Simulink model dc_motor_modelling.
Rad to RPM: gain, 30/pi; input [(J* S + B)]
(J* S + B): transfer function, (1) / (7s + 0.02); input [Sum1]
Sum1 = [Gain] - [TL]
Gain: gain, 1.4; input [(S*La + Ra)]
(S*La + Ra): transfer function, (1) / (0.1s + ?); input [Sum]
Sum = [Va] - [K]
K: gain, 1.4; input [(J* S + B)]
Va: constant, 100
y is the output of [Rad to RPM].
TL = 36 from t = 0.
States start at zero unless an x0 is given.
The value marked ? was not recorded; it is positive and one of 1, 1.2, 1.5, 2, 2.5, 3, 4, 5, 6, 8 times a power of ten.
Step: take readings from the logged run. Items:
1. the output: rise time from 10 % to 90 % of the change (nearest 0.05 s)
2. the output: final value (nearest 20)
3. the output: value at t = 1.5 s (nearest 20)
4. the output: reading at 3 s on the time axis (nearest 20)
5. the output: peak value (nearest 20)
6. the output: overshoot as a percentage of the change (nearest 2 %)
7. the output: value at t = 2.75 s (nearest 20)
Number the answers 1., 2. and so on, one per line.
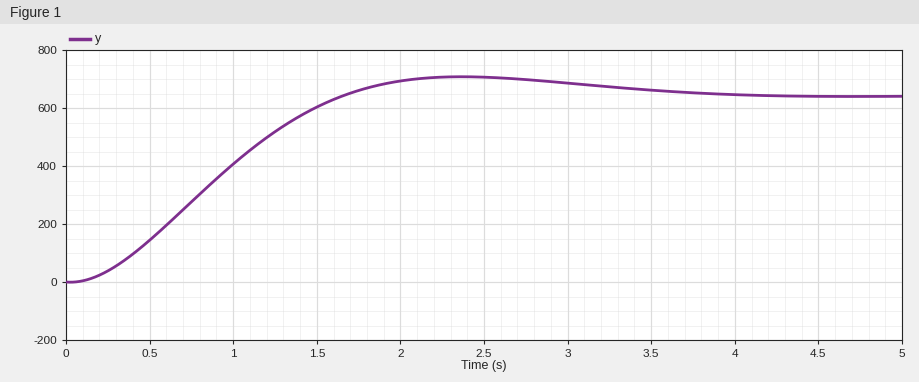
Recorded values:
1. 1.10 s
2. 640
3. 600
4. 680
5. 700
6. 10 %
7. 700
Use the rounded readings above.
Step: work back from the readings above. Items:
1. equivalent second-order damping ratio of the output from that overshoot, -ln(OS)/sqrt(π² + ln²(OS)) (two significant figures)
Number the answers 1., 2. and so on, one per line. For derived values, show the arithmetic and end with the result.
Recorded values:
1. ln(0.1) = -2.303; 2.303 / sqrt(9.870 + 5.302) = 0.59
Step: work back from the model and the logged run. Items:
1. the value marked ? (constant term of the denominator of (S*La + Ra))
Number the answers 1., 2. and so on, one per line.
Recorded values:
1. 0.2
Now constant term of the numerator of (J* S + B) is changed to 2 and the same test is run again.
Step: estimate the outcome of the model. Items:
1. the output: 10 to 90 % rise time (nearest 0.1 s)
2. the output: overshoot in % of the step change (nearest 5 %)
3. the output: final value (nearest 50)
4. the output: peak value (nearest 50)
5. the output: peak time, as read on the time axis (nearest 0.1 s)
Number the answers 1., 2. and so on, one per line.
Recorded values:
1. 0.6 s
2. 25 %
3. 650
4. 800
5. 1.5 s
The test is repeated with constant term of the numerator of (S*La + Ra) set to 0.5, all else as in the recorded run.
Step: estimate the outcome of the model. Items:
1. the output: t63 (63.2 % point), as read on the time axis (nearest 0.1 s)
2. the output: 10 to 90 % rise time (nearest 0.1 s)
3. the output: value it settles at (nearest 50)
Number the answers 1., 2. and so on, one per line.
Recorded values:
1. 1.7 s
2. 2.2 s
3. 600
